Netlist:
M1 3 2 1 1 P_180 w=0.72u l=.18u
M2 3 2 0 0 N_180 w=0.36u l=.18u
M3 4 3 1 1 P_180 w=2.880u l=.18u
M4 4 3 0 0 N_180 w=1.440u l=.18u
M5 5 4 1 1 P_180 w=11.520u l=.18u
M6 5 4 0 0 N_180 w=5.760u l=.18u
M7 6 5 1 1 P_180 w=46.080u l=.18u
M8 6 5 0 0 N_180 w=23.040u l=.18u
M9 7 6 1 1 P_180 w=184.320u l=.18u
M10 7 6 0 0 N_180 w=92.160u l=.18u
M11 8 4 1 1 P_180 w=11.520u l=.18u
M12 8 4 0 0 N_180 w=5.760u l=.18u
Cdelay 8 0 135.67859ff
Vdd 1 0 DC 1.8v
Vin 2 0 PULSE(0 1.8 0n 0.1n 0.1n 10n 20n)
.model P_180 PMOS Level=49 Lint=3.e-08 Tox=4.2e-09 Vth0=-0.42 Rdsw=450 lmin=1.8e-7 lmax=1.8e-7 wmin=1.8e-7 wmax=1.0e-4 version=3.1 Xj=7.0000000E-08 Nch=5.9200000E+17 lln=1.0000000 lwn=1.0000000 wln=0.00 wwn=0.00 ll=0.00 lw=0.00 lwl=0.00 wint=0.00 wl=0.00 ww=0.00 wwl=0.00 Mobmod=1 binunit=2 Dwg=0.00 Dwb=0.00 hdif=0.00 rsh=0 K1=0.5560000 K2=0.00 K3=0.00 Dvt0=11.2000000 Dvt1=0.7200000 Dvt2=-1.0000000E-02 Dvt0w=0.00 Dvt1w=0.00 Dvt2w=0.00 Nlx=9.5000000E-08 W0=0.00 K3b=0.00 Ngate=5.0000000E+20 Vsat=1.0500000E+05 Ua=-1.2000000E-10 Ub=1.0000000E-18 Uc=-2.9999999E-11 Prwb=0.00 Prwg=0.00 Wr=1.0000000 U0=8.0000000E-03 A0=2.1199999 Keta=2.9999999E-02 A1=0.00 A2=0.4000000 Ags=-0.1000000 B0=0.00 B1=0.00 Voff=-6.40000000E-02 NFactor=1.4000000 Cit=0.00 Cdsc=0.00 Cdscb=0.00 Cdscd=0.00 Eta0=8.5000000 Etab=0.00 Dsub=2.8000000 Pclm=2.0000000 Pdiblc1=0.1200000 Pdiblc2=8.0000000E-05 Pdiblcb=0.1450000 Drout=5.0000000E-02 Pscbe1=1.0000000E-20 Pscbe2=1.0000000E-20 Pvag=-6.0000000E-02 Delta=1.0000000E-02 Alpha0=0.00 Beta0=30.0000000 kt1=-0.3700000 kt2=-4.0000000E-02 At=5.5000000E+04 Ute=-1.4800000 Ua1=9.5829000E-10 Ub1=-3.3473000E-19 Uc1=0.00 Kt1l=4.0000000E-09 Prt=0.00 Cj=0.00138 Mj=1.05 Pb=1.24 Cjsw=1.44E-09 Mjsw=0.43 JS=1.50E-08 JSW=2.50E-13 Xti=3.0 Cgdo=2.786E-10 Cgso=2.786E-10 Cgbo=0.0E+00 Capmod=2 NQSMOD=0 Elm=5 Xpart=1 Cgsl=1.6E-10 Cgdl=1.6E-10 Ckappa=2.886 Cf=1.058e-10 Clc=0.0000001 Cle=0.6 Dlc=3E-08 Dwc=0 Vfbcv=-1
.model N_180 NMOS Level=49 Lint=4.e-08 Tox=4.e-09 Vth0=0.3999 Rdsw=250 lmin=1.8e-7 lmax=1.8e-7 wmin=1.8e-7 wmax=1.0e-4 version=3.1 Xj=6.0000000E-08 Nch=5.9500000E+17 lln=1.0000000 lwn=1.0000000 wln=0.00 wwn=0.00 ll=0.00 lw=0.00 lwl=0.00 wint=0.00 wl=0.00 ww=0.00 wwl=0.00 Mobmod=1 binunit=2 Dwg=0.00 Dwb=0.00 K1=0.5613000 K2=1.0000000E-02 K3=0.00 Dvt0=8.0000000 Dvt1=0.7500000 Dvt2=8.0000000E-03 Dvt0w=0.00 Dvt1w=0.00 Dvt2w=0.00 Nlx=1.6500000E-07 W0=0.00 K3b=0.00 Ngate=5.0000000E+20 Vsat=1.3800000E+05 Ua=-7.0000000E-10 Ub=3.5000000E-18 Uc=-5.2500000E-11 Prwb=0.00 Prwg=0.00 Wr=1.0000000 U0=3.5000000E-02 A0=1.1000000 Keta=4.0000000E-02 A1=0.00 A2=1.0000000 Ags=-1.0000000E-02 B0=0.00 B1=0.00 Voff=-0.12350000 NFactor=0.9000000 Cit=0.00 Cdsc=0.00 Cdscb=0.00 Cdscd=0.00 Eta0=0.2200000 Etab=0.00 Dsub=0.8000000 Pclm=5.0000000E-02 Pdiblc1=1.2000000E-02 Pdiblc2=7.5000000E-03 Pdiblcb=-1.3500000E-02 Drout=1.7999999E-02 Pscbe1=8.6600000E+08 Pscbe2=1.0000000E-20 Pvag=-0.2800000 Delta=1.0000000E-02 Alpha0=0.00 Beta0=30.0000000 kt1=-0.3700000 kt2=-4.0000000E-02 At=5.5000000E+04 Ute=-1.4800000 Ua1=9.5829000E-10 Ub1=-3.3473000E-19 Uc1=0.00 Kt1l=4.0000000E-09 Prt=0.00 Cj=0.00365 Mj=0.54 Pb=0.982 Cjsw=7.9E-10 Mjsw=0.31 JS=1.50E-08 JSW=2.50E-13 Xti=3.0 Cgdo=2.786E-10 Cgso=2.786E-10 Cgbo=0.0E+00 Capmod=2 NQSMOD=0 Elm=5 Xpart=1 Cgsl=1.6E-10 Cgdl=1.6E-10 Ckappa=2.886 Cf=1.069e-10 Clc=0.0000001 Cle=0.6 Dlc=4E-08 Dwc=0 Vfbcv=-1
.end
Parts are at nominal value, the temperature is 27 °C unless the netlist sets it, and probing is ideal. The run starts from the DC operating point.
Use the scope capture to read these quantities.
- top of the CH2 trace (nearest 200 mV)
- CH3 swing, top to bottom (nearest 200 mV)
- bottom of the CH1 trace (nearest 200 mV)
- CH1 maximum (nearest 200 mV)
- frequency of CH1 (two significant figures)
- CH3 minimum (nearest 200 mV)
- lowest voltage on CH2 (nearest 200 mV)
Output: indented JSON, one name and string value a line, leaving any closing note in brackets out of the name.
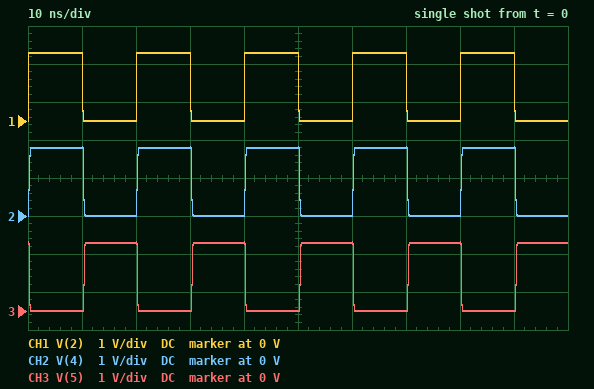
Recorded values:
{
  "top of the CH2 trace": "1.8 V",
  "CH3 swing, top to bottom": "1.8 V",
  "bottom of the CH1 trace": "0 V",
  "CH1 maximum": "1.8 V",
  "frequency of CH1": "50 MHz",
  "CH3 minimum": "0 V",
  "lowest voltage on CH2": "0 V"
}
